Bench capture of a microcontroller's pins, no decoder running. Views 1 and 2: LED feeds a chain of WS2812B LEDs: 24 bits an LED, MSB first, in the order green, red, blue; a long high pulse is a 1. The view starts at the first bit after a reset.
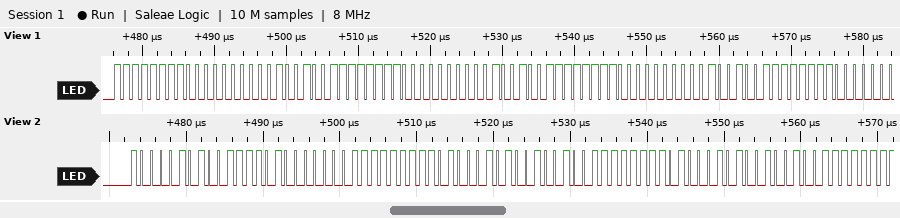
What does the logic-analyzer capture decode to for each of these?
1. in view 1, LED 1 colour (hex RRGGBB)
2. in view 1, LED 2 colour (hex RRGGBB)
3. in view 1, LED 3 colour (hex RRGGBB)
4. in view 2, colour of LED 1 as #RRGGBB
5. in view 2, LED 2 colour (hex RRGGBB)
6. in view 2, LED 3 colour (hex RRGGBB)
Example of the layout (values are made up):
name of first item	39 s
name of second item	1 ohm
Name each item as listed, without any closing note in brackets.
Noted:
in view 1, LED 1 colour	#00FF24
in view 1, LED 2 colour	#00FF24
in view 1, LED 3 colour	#00FF24
in view 2, colour of LED 1 as #RRGGBB	#3D8501
in view 2, LED 2 colour	#45FF24
in view 2, LED 3 colour	#45FF24
